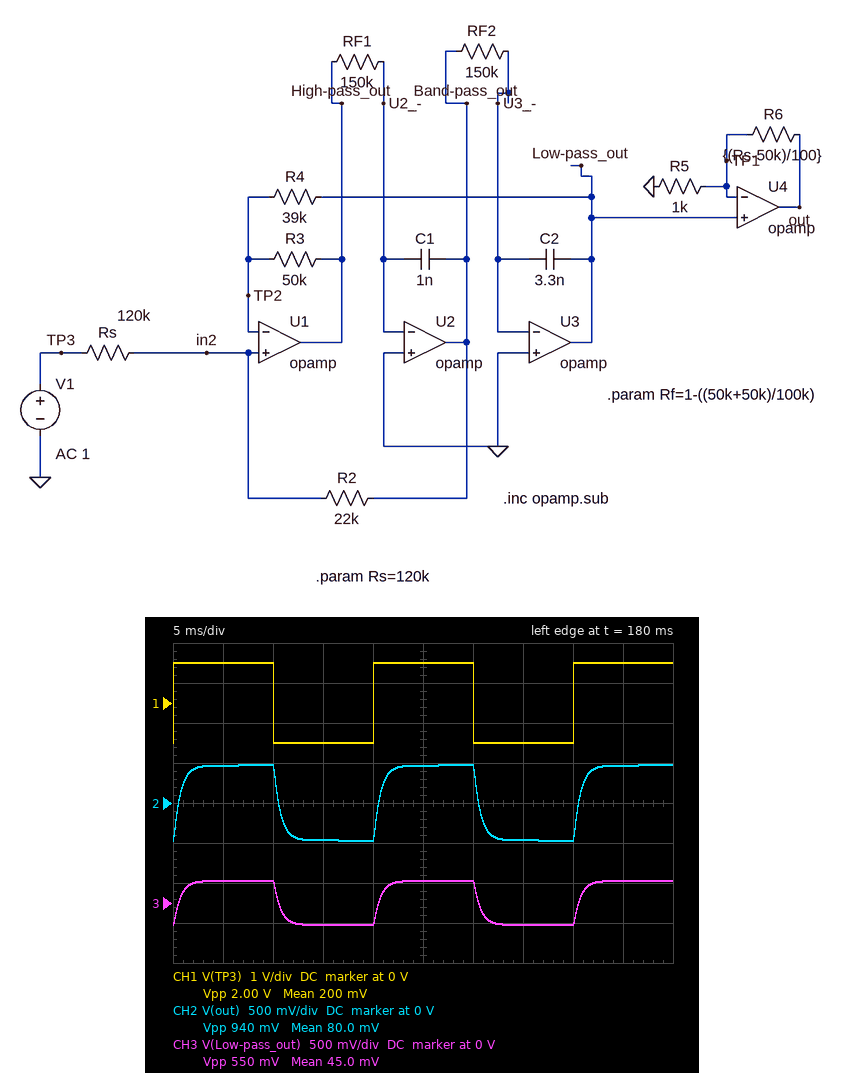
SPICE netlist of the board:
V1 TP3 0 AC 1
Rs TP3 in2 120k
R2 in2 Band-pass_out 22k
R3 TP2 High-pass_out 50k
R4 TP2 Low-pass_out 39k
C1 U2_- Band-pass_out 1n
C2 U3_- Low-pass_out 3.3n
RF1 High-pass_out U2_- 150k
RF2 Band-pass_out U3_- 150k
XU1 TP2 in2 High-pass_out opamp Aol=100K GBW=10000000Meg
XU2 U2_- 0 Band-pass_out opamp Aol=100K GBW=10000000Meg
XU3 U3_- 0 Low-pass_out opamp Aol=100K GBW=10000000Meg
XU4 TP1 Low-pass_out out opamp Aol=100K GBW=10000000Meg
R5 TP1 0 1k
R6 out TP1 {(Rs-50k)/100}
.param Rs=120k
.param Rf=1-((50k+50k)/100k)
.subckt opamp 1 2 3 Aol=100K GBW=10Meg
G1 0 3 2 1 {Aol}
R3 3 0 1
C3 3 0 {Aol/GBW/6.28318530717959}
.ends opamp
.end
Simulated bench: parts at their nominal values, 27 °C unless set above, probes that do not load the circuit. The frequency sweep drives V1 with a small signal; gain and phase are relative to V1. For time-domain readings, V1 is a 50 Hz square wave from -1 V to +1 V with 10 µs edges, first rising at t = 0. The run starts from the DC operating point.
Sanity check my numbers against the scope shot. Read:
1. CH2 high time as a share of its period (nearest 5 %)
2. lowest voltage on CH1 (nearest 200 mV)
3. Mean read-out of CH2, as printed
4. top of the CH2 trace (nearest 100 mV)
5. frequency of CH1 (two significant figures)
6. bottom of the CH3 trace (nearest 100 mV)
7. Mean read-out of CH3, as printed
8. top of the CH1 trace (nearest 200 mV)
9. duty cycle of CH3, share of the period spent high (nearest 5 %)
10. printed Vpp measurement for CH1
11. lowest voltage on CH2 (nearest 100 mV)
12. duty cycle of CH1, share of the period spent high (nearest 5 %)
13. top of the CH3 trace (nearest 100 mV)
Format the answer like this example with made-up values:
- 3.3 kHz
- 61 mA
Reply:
- 50 %
- -1.0 V
- 80.0 mV
- 500 mV
- 50 Hz
- -300 mV
- 45.0 mV
- 1.0 V
- 50 %
- 2.00 V
- -500 mV
- 50 %
- 300 mV
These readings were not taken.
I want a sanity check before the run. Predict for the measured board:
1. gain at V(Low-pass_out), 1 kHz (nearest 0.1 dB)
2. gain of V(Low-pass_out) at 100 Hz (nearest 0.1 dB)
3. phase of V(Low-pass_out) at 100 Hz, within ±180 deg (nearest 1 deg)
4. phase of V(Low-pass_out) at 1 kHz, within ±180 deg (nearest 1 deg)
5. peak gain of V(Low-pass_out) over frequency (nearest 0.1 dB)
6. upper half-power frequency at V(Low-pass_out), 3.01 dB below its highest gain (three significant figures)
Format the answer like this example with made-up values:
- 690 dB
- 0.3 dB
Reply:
- -24.9 dB
- -11.9 dB
- -26 deg
- -105 deg
- -11.2 dB
- 238 Hz
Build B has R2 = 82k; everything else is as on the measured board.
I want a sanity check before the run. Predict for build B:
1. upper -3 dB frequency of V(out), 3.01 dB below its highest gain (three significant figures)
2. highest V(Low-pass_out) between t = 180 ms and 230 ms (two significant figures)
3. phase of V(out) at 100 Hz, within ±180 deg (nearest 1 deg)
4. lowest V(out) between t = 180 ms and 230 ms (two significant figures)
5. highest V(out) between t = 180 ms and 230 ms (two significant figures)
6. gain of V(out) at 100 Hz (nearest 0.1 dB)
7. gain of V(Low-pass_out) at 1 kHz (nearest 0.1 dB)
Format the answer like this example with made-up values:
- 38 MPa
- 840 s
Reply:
- 378 Hz
- 720 mV
- -19 deg
- -1.2 V
- 1.2 V
- 1.5 dB
- -13.8 dB
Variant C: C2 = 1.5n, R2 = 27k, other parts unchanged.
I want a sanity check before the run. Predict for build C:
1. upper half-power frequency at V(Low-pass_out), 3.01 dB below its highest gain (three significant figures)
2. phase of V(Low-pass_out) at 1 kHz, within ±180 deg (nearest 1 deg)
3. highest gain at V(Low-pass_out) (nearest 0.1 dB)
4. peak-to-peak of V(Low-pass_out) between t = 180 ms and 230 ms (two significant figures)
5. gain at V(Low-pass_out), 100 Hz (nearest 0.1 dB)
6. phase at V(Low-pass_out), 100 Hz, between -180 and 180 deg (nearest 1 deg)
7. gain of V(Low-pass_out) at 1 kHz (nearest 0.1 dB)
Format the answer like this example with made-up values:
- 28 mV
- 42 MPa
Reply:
- 625 Hz
- -91 deg
- -9.7 dB
- 650 mV
- -9.8 dB
- -12 deg
- -16.0 dB
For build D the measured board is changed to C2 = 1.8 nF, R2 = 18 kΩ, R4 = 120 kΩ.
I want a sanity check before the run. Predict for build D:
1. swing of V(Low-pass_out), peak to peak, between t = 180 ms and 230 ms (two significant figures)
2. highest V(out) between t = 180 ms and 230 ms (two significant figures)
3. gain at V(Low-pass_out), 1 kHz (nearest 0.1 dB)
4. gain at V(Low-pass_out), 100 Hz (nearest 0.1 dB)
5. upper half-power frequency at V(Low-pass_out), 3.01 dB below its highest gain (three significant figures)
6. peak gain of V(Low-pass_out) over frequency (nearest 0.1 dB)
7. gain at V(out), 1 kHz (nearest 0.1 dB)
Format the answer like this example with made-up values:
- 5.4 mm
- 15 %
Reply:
- 890 mV
- 750 mV
- -22.3 dB
- -7.8 dB
- 234 Hz
- -7.1 dB
- -17.7 dB
